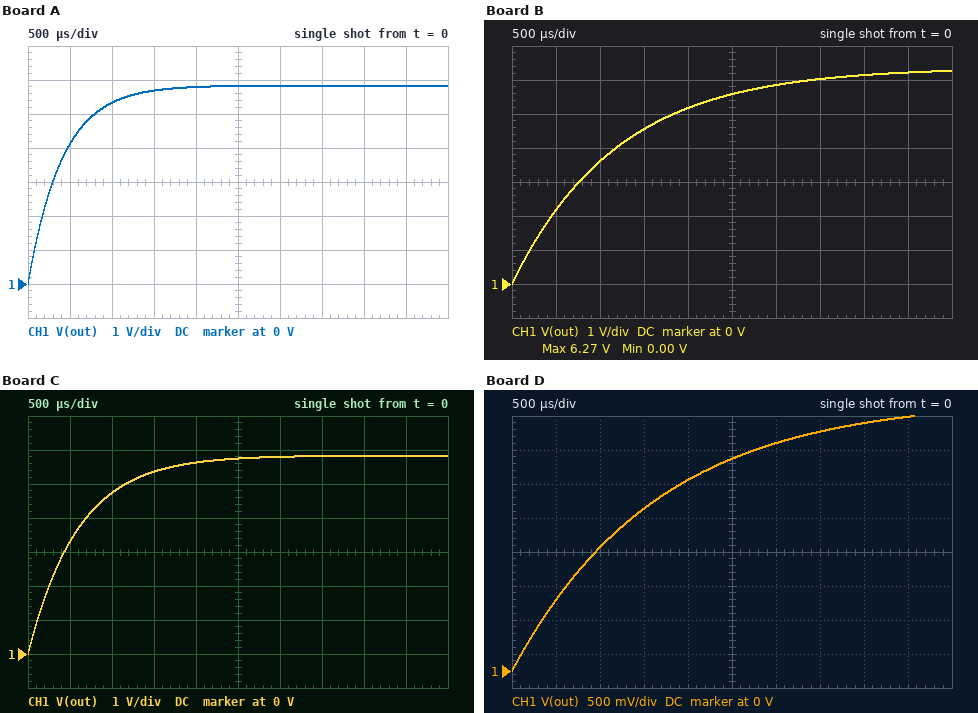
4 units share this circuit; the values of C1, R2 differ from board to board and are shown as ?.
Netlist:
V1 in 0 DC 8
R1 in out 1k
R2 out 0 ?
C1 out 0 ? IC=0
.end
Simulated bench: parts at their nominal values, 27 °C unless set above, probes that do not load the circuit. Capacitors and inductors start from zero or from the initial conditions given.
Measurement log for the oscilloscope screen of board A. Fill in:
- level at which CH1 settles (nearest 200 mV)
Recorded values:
5.8 V
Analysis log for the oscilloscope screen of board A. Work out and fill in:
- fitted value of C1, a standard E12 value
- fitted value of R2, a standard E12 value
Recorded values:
560 nF
2.7 kΩ
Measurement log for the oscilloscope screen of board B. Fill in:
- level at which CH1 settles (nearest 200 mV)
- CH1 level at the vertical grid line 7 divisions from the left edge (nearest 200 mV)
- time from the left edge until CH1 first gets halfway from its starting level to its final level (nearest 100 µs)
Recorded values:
6.2 V
6.0 V
800 µs
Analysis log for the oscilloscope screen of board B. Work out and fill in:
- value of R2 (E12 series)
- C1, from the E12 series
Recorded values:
3.9 kΩ
1.5 µF
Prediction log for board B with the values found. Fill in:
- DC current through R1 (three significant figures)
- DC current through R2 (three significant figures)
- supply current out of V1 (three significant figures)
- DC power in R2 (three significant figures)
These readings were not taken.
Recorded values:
1.63 mA
1.63 mA
1.63 mA
10.4 mW
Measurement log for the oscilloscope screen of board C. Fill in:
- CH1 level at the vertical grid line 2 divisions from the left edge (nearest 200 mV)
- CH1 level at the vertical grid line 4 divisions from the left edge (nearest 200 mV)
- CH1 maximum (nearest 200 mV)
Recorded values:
4.8 V
5.6 V
5.8 V
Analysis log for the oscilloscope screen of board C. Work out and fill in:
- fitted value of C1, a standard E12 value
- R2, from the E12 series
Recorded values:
820 nF
2.7 kΩ
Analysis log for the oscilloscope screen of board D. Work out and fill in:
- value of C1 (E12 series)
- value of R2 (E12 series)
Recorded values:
3.3 µF
1 kΩ
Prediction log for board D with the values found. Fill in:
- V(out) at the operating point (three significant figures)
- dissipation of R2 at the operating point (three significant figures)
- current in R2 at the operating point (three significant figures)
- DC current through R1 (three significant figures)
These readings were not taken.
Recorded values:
4.00 V
16.0 mW
4.00 mA
4.00 mA
